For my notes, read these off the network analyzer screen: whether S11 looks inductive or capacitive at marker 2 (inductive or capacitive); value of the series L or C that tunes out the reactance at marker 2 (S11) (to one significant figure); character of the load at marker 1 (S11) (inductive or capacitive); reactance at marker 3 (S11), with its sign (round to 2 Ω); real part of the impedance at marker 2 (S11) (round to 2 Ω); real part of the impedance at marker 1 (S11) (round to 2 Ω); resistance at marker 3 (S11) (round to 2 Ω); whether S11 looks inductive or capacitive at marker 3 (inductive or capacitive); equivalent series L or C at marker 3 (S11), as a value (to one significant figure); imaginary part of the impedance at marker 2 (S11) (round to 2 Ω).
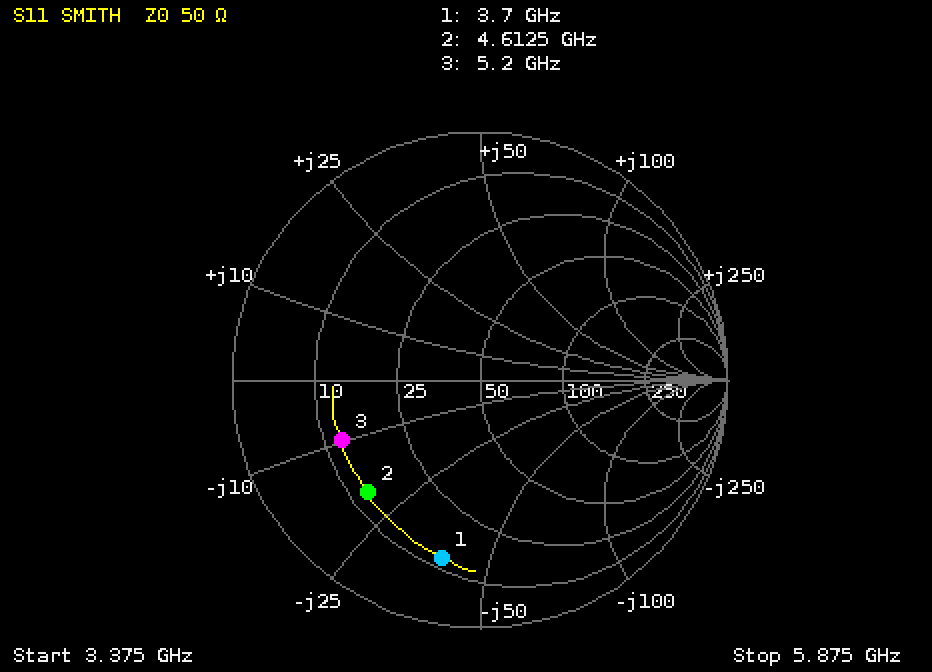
capacitive
700 pH
capacitive
-10 Ω
12 Ω
12 Ω
12 Ω
capacitive
3 pF
-20 Ω
